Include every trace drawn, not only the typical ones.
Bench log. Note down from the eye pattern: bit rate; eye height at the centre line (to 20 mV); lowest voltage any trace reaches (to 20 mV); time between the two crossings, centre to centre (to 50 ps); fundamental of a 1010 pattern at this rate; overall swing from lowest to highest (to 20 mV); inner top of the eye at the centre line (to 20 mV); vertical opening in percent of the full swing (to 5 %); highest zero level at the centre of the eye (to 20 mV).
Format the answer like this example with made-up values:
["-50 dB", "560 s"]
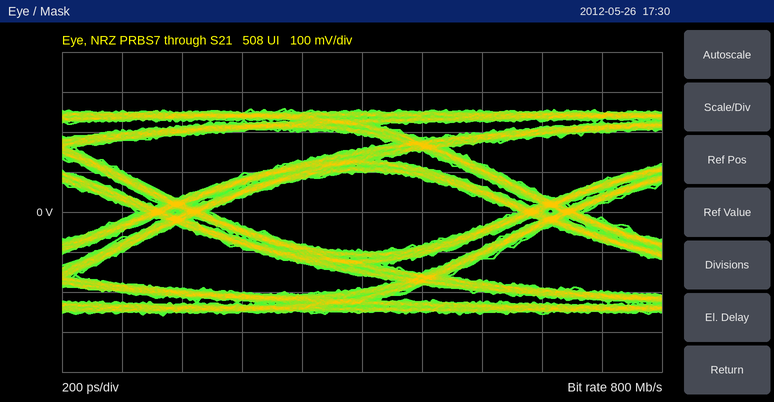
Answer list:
["800 Mb/s", "200 mV", "-260 mV", "1.25 ns", "400 MHz", "520 mV", "100 mV", "40 %", "-100 mV"]
